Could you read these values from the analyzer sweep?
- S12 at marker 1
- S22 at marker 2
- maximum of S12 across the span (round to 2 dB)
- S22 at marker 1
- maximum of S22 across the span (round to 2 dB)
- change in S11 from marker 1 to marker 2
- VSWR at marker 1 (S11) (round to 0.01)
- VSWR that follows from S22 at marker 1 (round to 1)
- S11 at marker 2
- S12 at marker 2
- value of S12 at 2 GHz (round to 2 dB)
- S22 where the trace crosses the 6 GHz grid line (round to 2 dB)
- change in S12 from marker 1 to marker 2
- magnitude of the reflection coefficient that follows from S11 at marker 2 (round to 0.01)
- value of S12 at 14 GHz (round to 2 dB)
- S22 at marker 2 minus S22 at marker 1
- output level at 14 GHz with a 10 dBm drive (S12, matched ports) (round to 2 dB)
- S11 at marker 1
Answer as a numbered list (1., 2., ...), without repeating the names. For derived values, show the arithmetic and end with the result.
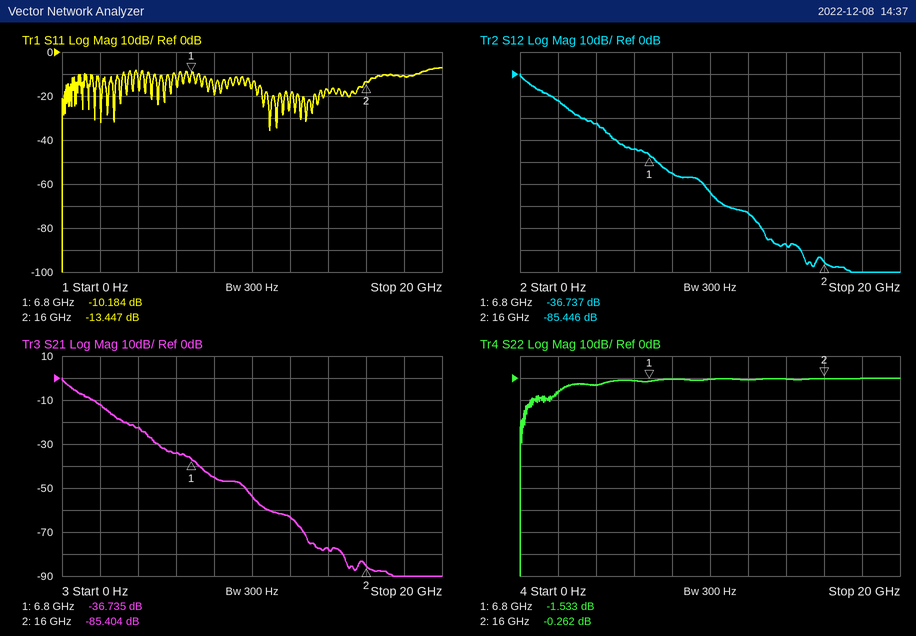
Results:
1. -36.737 dB
2. -0.262 dB
3. 0 dB
4. -1.533 dB
5. 0 dB
6. -13.447 − (-10.184) = -3.263 dB
7. (1 + 0.3096)/(1 − 0.3096) ≈ 1.90
8. (1 + 0.8382)/(1 − 0.8382) ≈ 11
9. -13.447 dB
10. -85.446 dB
11. -12 dB
12. -2 dB
13. -85.446 − (-36.737) = -48.709 dB
14. 10^(-13.447/20) ≈ 0.21
15. -78 dB
16. -0.262 − (-1.533) = 1.271 dB
17. 10 dBm + (-78 dB) = -68 dBm
18. -10.184 dB
